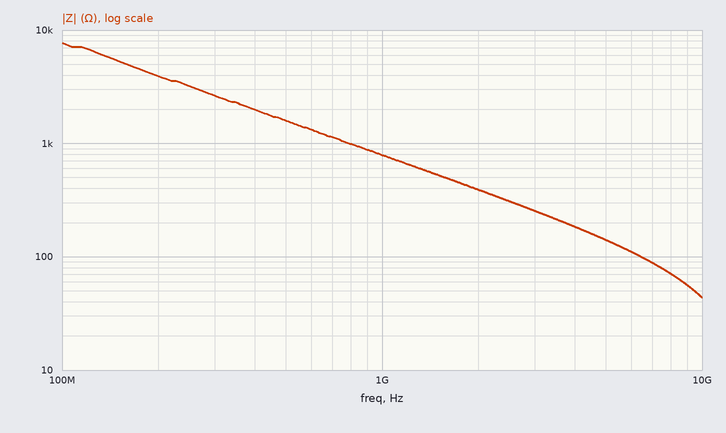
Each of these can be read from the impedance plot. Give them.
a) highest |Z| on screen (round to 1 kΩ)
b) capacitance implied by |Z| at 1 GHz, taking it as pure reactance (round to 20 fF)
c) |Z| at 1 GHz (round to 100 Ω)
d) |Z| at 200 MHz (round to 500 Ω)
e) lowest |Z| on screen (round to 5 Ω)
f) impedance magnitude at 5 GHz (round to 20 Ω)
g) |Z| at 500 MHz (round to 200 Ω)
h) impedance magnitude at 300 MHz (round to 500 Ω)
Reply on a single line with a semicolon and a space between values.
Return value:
8 kΩ; 200 fF; 800 Ω; 4.0 kΩ; 45 Ω; 140 Ω; 1.6 kΩ; 2.5 kΩ
